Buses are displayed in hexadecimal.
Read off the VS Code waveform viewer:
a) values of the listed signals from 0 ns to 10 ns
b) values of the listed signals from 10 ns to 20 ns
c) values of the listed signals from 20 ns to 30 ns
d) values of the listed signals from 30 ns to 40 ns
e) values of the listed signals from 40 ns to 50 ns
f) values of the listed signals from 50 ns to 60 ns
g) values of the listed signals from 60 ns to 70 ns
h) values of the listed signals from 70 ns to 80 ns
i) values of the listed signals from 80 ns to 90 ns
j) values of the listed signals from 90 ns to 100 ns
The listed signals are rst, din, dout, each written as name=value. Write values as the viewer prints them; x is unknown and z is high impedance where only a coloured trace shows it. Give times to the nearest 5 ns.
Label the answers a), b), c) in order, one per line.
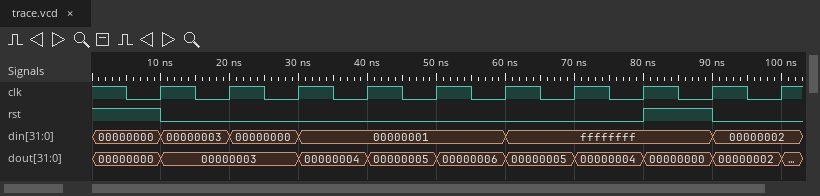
a) rst=1, din=00000000, dout=00000000
b) rst=0, din=00000003, dout=00000003
c) rst=0, din=00000000, dout=00000003
d) rst=0, din=00000001, dout=00000004
e) rst=0, din=00000001, dout=00000005
f) rst=0, din=00000001, dout=00000006
g) rst=0, din=ffffffff, dout=00000005
h) rst=0, din=ffffffff, dout=00000004
i) rst=1, din=ffffffff, dout=00000000
j) rst=0, din=00000002, dout=00000002
